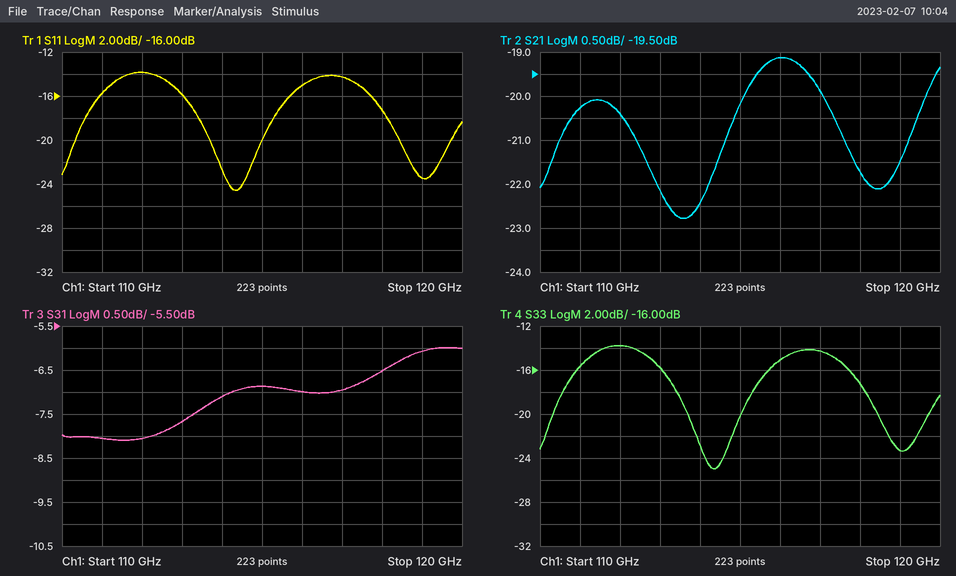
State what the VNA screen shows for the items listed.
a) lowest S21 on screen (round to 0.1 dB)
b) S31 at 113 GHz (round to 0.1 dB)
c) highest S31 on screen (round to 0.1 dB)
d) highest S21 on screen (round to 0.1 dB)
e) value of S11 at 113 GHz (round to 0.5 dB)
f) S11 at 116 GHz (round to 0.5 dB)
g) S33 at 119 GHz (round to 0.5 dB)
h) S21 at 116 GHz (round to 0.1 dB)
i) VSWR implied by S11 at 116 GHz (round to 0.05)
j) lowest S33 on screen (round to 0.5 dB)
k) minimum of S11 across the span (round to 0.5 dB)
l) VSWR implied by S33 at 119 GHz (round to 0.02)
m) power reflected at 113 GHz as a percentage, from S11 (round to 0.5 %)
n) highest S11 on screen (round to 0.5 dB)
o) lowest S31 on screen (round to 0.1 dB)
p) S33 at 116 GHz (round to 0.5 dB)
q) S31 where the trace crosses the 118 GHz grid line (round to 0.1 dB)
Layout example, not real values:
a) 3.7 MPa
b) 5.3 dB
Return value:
a) -22.8 dB
b) -7.7 dB
c) -6.0 dB
d) -19.1 dB
e) -16.0 dB
f) -15.0 dB
g) -23.5 dB
h) -19.1 dB
i) 1.45
j) -25.0 dB
k) -24.5 dB
l) 1.14
m) 2.5 %
n) -14.0 dB
o) -8.1 dB
p) -15.0 dB
q) -6.5 dB
